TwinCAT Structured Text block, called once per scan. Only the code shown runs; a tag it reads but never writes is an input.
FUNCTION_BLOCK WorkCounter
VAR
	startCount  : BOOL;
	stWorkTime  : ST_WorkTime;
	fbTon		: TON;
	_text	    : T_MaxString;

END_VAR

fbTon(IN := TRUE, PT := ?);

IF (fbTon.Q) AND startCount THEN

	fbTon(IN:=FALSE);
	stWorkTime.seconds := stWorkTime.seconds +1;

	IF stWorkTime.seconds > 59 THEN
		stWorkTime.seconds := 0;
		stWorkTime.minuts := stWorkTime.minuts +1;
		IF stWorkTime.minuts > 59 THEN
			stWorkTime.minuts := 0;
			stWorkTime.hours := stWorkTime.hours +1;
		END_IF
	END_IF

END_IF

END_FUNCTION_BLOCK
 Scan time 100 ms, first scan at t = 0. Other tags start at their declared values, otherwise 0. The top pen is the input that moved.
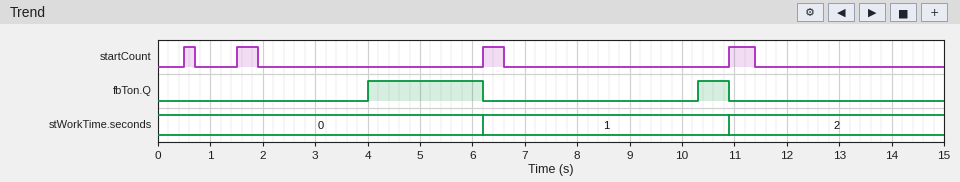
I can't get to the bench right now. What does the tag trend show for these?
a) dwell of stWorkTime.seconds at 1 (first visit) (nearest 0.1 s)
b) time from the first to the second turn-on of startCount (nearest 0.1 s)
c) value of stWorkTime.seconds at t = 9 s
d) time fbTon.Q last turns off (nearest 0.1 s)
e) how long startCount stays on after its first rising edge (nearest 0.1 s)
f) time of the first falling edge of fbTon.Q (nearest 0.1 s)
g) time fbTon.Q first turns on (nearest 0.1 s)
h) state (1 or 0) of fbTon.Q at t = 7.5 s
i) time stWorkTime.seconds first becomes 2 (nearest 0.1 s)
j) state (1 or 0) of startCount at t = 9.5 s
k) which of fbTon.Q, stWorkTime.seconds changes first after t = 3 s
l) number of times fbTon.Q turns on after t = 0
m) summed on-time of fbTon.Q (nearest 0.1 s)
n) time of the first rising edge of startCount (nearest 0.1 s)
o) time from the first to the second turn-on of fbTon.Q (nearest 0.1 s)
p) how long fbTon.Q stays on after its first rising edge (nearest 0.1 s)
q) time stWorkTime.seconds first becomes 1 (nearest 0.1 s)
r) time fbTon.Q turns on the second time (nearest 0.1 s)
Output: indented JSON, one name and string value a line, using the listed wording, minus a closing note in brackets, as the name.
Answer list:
{
  "dwell of stWorkTime.seconds at 1 (first visit)": "4.7 s",
  "time from the first to the second turn-on of startCount": "1.0 s",
  "value of stWorkTime.seconds at t = 9 s": "1",
  "time fbTon.Q last turns off": "10.9 s",
  "how long startCount stays on after its first rising edge": "0.2 s",
  "time of the first falling edge of fbTon.Q": "6.2 s",
  "time fbTon.Q first turns on": "4.0 s",
  "state (1 or 0) of fbTon.Q at t = 7.5 s": "0",
  "time stWorkTime.seconds first becomes 2": "10.9 s",
  "state (1 or 0) of startCount at t = 9.5 s": "0",
  "which of fbTon.Q, stWorkTime.seconds changes first after t = 3 s": "fbTon.Q",
  "number of times fbTon.Q turns on after t = 0": "2",
  "summed on-time of fbTon.Q": "2.8 s",
  "time of the first rising edge of startCount": "0.5 s",
  "time from the first to the second turn-on of fbTon.Q": "6.3 s",
  "how long fbTon.Q stays on after its first rising edge": "2.2 s",
  "time stWorkTime.seconds first becomes 1": "6.2 s",
  "time fbTon.Q turns on the second time": "10.3 s"
}
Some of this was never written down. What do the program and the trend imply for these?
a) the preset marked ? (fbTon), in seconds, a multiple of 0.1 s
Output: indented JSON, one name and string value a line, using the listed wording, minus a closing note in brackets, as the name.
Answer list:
{
  "the preset marked ? (fbTon), in seconds, a multiple of 0.1 s": "4.0 s"
}
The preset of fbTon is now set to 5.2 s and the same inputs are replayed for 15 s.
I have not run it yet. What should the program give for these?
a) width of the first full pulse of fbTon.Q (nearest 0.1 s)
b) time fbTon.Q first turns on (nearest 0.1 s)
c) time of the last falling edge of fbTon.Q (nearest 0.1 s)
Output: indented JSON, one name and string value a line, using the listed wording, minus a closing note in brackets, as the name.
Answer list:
{
  "width of the first full pulse of fbTon.Q": "1.0 s",
  "time fbTon.Q first turns on": "5.2 s",
  "time of the last falling edge of fbTon.Q": "6.2 s"
}
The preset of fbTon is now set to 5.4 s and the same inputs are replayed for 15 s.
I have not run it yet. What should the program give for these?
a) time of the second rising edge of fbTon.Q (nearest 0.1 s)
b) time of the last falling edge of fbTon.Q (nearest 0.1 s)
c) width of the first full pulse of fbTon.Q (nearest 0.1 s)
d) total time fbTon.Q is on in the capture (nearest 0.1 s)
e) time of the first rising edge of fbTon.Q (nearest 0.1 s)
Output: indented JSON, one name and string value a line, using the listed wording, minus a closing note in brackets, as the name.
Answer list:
{
  "time of the second rising edge of fbTon.Q": "11.7 s",
  "time of the last falling edge of fbTon.Q": "6.2 s",
  "width of the first full pulse of fbTon.Q": "0.8 s",
  "total time fbTon.Q is on in the capture": "4.1 s",
  "time of the first rising edge of fbTon.Q": "5.4 s"
}
